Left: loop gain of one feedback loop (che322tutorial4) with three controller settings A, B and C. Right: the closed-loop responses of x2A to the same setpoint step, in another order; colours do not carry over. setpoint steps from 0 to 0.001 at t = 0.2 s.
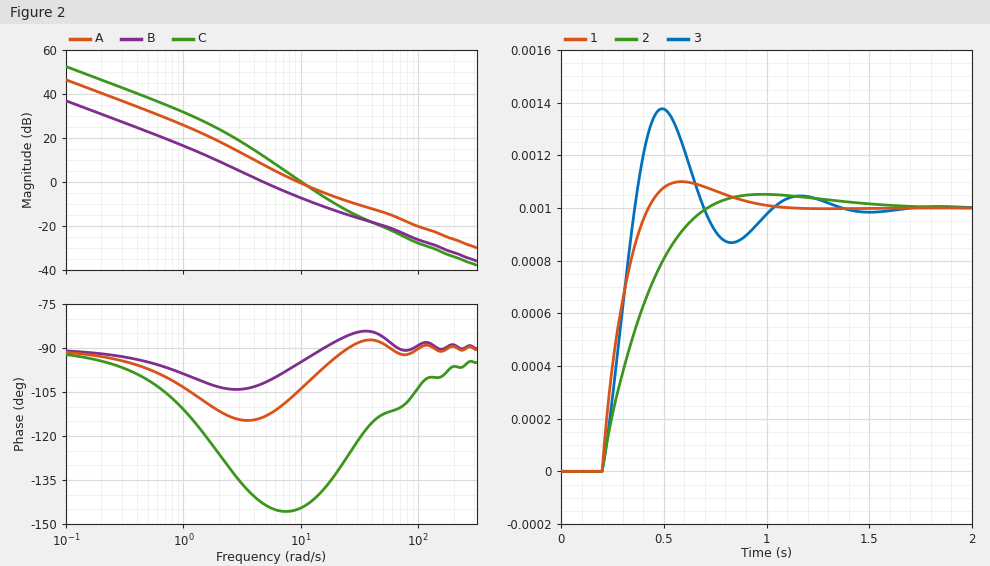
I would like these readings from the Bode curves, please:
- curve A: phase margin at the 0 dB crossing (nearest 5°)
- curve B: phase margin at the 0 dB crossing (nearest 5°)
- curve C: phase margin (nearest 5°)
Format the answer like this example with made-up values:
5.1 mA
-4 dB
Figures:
75°
80°
35°
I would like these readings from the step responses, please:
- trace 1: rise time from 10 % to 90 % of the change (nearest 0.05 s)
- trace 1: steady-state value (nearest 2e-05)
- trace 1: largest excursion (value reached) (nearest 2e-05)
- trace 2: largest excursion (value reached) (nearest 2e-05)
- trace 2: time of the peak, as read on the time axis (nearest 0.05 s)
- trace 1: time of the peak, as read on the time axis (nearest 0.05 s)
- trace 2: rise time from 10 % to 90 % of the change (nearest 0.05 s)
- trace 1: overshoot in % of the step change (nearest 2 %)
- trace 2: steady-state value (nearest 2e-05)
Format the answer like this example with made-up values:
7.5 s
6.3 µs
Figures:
0.15 s
0.00100
0.00110
0.00106
1.00 s
0.60 s
0.35 s
10 %
0.00100
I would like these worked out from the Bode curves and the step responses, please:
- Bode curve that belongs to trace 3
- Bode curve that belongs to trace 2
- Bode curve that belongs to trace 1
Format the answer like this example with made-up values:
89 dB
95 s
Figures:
C
B
A
